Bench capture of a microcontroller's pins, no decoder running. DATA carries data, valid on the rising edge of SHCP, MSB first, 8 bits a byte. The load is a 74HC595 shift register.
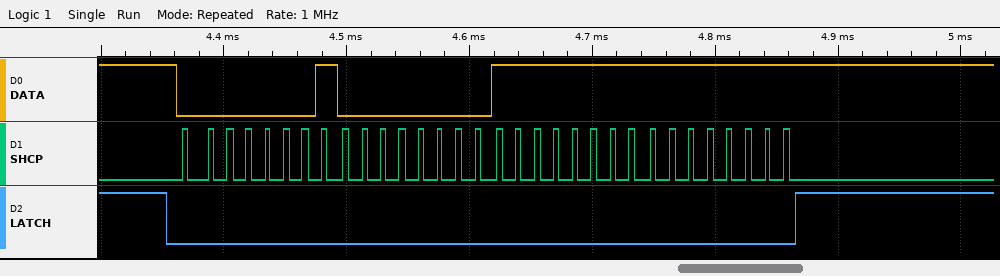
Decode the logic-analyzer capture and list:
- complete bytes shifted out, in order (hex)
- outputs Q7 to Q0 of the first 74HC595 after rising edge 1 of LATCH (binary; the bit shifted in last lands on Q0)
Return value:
01 00 FF FF
11111111
